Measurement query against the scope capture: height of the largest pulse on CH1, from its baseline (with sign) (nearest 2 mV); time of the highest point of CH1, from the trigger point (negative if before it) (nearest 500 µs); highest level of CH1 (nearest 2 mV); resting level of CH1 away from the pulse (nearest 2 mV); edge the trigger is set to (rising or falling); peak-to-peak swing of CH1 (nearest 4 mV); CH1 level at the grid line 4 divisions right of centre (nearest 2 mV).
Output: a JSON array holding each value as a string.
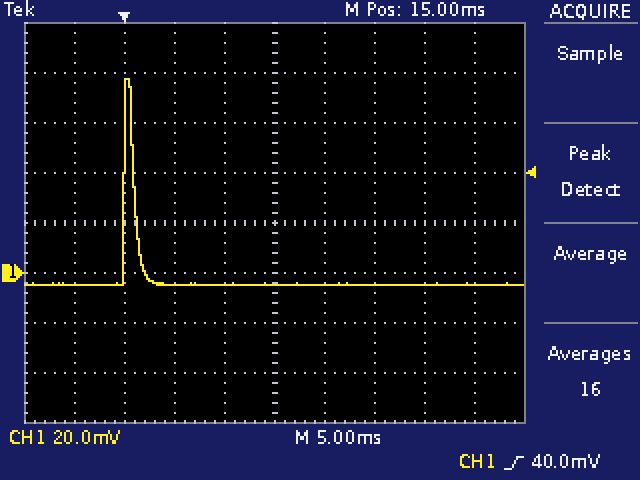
["+82 mV", "+500 µs", "78 mV", "-4 mV", "rising", "84 mV", "-4 mV"]
